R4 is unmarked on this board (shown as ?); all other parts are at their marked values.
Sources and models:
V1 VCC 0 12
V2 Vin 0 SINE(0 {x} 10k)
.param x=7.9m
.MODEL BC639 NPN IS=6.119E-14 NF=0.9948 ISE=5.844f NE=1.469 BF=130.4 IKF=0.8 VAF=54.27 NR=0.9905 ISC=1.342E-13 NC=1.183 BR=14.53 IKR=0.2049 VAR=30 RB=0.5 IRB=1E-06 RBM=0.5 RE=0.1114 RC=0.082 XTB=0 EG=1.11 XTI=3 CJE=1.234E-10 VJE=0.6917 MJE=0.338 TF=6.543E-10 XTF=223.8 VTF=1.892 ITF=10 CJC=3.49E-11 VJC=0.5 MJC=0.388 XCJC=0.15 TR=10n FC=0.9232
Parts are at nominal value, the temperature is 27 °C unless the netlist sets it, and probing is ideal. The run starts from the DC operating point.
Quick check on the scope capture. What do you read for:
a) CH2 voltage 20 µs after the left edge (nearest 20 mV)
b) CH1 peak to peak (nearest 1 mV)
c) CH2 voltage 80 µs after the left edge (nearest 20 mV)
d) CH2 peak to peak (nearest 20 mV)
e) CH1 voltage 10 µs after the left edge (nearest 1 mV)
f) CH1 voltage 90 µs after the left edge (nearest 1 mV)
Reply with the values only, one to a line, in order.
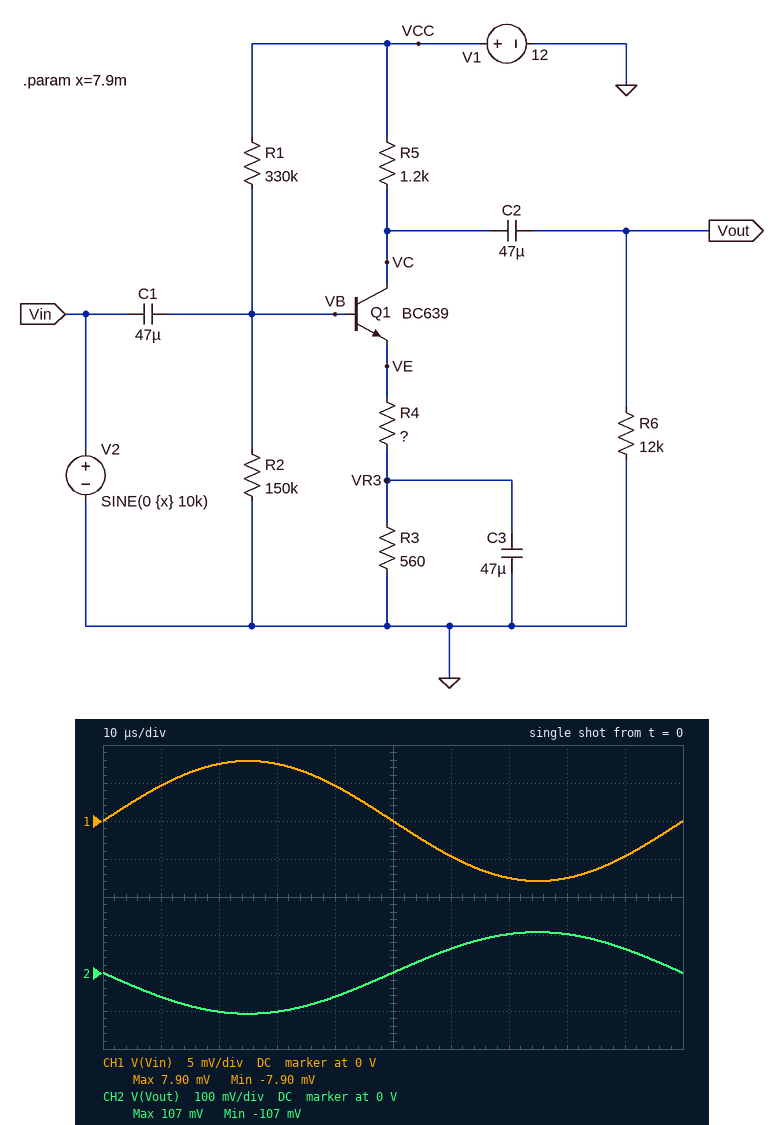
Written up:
-100 mV
16 mV
100 mV
220 mV
5 mV
-5 mV
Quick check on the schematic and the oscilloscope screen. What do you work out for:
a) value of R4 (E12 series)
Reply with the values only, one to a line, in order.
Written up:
68 Ω
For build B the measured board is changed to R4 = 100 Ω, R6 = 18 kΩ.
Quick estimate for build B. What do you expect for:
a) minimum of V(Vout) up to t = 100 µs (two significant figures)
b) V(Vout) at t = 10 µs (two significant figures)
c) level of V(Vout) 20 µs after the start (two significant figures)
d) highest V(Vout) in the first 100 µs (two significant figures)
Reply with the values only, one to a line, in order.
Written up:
-79 mV
-46 mV
-75 mV
79 mV
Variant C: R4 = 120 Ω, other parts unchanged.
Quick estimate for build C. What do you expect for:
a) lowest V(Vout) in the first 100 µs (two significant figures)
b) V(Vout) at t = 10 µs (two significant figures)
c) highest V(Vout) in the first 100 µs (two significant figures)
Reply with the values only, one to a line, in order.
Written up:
-65 mV
-38 mV
65 mV
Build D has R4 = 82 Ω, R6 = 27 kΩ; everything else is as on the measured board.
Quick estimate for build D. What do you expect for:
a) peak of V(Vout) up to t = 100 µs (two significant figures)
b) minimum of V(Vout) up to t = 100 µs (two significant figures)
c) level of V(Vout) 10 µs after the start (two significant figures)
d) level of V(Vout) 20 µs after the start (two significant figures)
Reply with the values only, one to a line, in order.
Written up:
96 mV
-96 mV
-56 mV
-91 mV
